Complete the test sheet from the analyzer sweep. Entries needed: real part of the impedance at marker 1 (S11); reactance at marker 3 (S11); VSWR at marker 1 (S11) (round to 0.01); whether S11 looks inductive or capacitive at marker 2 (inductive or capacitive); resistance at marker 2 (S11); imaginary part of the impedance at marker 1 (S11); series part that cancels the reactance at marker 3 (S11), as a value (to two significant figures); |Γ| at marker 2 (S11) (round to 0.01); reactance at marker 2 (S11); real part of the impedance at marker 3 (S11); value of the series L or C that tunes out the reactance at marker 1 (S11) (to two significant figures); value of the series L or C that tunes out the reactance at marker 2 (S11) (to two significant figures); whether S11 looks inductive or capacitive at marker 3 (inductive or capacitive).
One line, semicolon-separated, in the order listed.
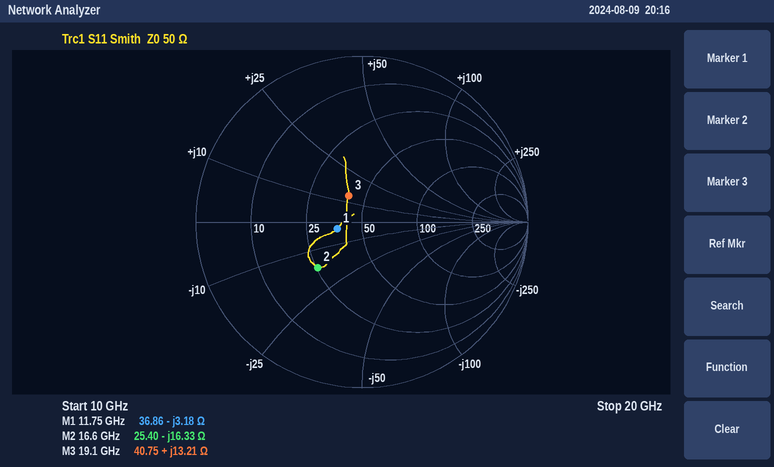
36.86 Ω; +13.21 Ω; 1.37; capacitive; 25.40 Ω; -3.18 Ω; 630 fF; 0.38; -16.33 Ω; 40.75 Ω; 43 pH; 160 pH; inductive
